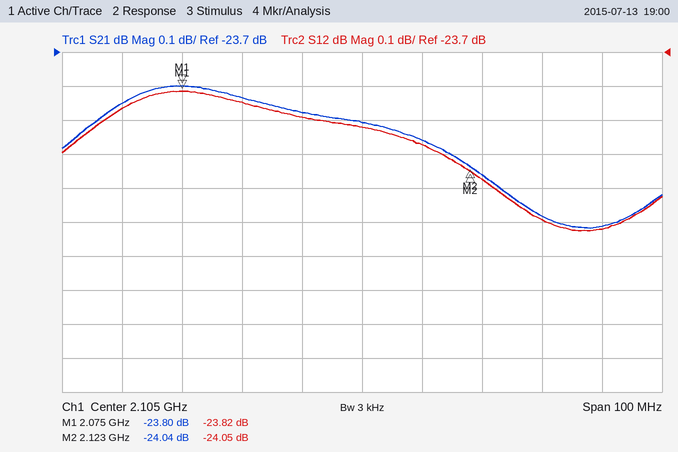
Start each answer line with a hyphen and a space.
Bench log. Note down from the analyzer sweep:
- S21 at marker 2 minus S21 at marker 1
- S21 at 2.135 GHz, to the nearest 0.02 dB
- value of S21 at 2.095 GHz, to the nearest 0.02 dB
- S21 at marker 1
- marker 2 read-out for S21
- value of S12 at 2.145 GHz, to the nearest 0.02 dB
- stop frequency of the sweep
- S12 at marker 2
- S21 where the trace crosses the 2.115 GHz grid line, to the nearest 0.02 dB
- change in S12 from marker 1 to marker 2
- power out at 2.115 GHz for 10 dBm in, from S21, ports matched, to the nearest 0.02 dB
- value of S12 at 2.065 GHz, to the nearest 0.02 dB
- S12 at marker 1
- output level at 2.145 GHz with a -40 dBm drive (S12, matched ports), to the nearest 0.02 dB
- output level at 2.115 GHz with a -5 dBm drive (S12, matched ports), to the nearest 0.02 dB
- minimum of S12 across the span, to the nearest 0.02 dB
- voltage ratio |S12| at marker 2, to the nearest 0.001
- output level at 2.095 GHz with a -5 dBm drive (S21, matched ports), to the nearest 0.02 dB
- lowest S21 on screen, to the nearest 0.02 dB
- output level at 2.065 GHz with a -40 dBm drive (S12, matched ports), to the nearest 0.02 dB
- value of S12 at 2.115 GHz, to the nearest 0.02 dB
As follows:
- -0.24 dB
- -24.18 dB
- -23.88 dB
- -23.80 dB
- -24.04 dB
- -24.22 dB
- 2.155 GHz
- -24.05 dB
- -23.96 dB
- -0.23 dB
- -13.96 dBm
- -23.86 dB
- -23.82 dB
- -64.22 dBm
- -28.98 dBm
- -24.22 dB
- 0.063
- -28.88 dBm
- -24.22 dB
- -63.86 dBm
- -23.98 dB
